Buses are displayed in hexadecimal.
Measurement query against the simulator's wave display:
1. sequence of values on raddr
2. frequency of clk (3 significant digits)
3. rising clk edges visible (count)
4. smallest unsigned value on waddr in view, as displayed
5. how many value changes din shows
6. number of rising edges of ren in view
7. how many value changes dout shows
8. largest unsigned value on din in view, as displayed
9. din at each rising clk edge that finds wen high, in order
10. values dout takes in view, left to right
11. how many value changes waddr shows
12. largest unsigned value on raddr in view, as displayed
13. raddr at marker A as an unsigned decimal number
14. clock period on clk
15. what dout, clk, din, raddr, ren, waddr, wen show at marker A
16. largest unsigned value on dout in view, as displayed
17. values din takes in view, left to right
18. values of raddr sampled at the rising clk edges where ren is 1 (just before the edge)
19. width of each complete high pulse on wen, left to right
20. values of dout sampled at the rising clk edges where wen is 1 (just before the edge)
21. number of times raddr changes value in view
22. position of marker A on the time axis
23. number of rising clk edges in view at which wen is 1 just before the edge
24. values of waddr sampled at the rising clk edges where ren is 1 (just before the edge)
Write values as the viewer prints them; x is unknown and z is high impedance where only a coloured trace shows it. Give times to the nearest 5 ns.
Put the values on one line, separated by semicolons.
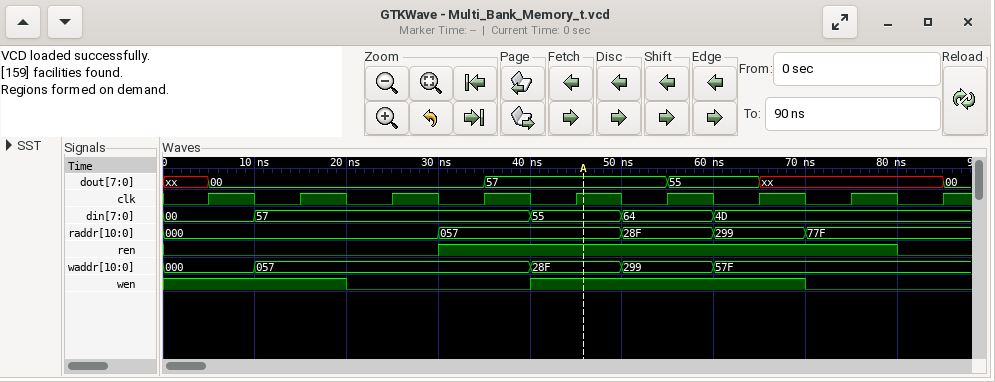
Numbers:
000, 057, 28F, 299, 77F; 100 MHz; 9; 000; 4; 1; 5; 64; 00, 57, 55, 64, 4D; xx, 00, 57, 55, xx, 00; 4; 77F; 87; 10 ns; dout=57, clk=1, din=55, raddr=057, ren=1, waddr=28F, wen=1; 57; 00, 57, 55, 64, 4D; 057, 057, 28F, 299, 77F; 30 ns; xx, 00, 57, 57, 55; 4; 45 ns; 5; 057, 28F, 299, 57F, 57F
